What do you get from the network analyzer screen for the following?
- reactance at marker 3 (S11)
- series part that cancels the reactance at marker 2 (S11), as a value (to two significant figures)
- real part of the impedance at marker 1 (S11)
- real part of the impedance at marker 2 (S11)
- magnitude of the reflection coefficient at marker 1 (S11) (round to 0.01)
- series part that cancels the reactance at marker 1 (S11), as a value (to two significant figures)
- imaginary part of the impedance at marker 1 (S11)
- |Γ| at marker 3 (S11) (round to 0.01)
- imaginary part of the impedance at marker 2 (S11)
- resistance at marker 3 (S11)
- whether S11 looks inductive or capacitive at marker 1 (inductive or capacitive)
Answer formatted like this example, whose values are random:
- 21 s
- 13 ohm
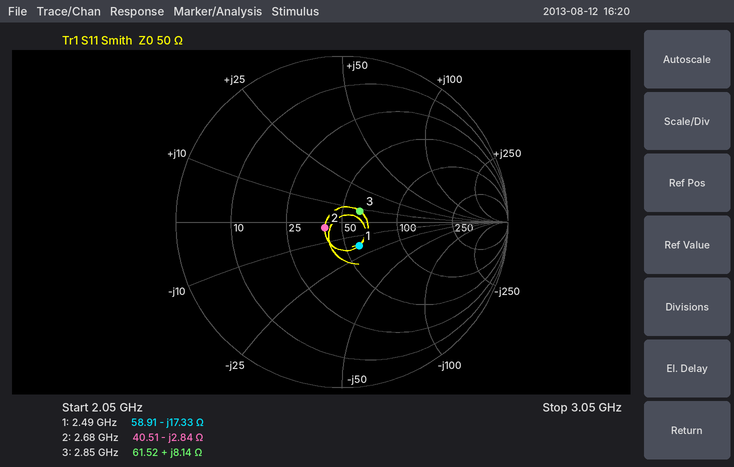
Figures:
- +8.14 Ω
- 170 pH
- 58.91 Ω
- 40.51 Ω
- 0.18
- 1.1 nH
- -17.33 Ω
- 0.13
- -2.84 Ω
- 61.52 Ω
- capacitive
